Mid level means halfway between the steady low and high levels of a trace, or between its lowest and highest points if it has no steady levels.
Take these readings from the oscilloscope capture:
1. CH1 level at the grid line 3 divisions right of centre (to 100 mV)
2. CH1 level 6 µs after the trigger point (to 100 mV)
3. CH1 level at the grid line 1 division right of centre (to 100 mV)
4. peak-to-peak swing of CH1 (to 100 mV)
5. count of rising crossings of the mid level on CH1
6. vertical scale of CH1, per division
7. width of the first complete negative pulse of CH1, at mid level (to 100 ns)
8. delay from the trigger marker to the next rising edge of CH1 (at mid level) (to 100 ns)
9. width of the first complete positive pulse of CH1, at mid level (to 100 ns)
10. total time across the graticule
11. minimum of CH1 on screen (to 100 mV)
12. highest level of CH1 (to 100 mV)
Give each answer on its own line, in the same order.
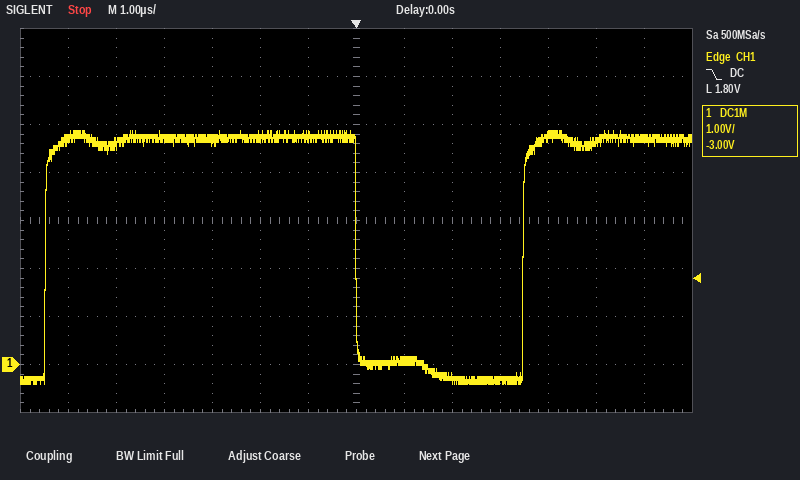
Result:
-300 mV
4.7 V
100 mV
5.3 V
2
1 V
3.5 µs
3.5 µs
6.5 µs
14 µs
-400 mV
4.9 V
